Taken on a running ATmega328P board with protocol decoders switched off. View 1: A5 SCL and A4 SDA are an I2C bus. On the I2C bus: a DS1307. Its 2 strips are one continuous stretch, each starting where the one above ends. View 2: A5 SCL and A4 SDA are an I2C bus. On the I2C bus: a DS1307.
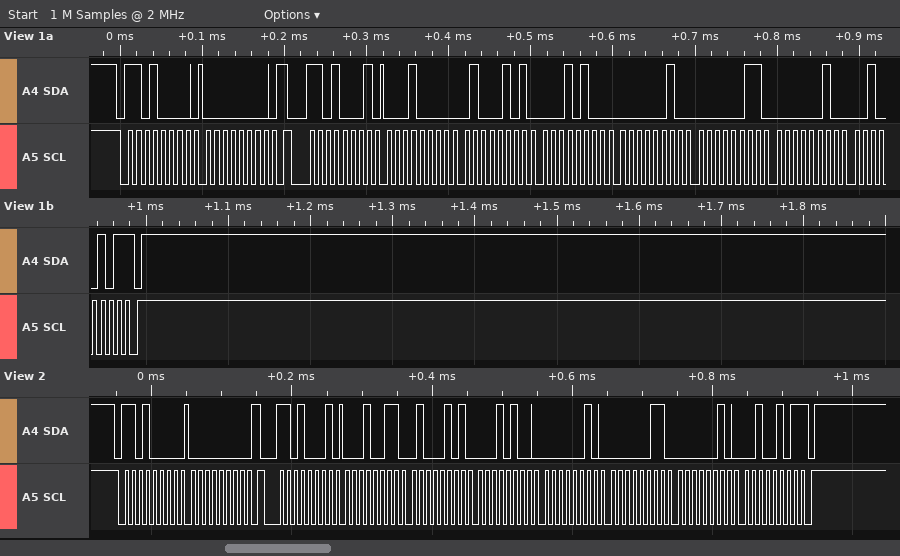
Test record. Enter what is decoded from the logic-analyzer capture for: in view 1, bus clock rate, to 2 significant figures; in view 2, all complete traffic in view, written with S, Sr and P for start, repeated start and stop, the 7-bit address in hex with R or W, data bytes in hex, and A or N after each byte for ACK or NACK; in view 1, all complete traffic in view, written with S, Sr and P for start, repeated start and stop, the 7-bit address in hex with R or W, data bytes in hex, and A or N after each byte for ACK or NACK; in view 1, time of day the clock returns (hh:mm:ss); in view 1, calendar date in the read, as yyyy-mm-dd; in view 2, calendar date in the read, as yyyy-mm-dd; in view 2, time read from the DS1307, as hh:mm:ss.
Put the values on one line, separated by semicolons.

100 kHz; S 68W A 00 A Sr 68R A 13 A 45 A 14 A 02 A 03 A 02 A 25 N P; S 68W A 00 A Sr 68R A 10 A 45 A 14 A 02 A 03 A 02 A 25 N P; 14:45:10; 2025-02-03; 2025-02-03; 14:45:13
